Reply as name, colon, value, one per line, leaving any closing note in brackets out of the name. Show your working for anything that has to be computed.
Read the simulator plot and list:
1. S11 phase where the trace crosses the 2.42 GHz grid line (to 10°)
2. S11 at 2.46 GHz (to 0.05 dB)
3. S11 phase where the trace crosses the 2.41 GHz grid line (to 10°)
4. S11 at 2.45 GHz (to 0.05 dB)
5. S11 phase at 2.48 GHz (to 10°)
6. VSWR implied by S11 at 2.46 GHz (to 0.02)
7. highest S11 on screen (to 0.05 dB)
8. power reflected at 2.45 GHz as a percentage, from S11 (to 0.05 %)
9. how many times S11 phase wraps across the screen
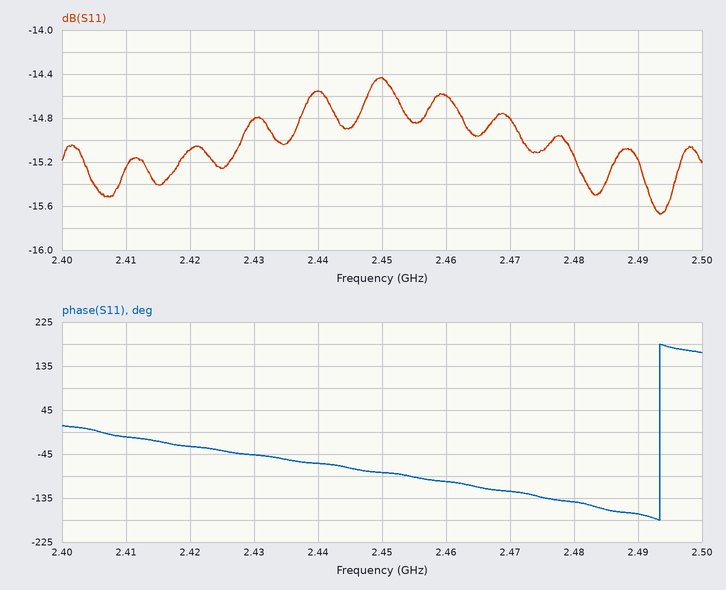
S11 phase where the trace crosses the 2.42 GHz grid line: -30°
S11 at 2.46 GHz: -14.60 dB
S11 phase where the trace crosses the 2.41 GHz grid line: -10°
S11 at 2.45 GHz: -14.45 dB
S11 phase at 2.48 GHz: -140°
VSWR implied by S11 at 2.46 GHz: |Γ| = 10^(-14.6/20) = 0.1862; VSWR = (1 + 0.1862)/(1 − 0.1862) ≈ 1.46
highest S11 on screen: -14.45 dB
power reflected at 2.45 GHz as a percentage, from S11: 10^(-14.45/10) ≈ 3.59 %, so 3.60 % to the nearest 0.05 %
how many times S11 phase wraps across the screen: 1
